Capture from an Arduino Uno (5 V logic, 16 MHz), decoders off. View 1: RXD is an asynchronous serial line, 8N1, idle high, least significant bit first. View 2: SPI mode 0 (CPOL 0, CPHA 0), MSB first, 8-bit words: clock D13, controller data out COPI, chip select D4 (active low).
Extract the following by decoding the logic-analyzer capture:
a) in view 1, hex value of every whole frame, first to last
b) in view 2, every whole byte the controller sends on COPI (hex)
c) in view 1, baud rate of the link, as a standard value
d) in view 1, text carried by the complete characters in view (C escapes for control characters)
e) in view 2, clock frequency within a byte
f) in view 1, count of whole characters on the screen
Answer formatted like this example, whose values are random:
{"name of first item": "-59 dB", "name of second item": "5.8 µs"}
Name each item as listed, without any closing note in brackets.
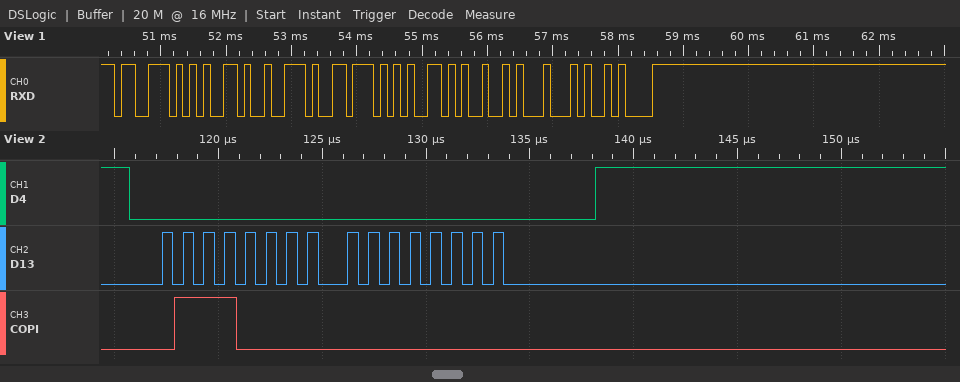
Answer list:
{"in view 1, hex value of every whole frame, first to last": "73 65 72 76 65 49 44 0A", "in view 2, every whole byte the controller sends on COPI": "70 00", "in view 1, baud rate of the link, as a standard value": "9600 baud", "in view 1, text carried by the complete characters in view": "\"serveID\\n\"", "in view 2, clock frequency within a byte": "1 MHz", "in view 1, count of whole characters on the screen": "8"}
